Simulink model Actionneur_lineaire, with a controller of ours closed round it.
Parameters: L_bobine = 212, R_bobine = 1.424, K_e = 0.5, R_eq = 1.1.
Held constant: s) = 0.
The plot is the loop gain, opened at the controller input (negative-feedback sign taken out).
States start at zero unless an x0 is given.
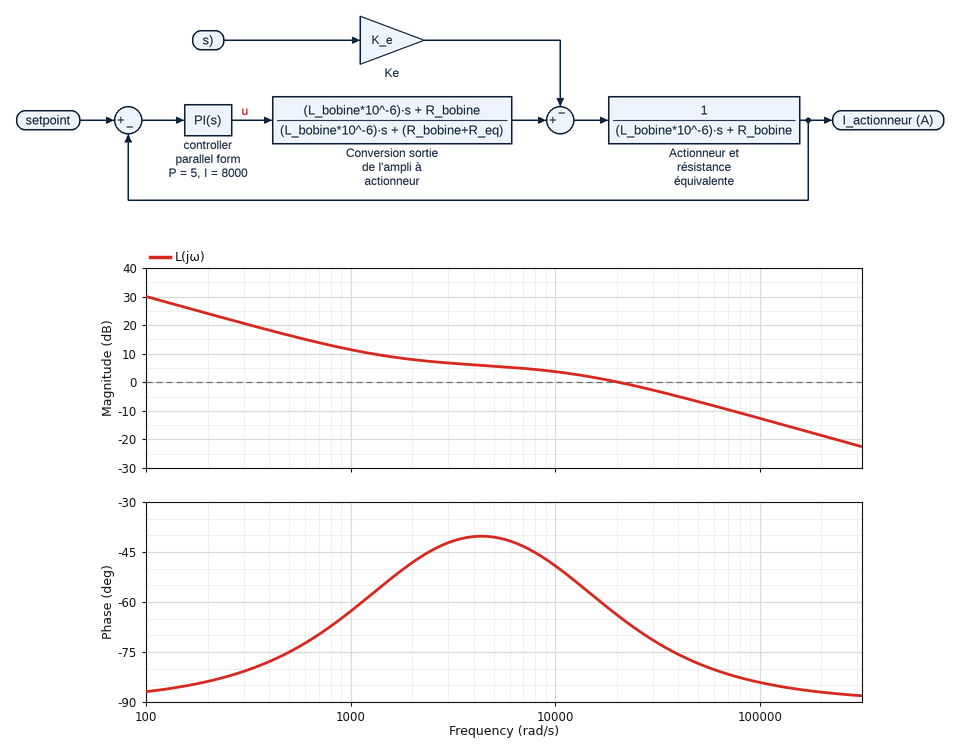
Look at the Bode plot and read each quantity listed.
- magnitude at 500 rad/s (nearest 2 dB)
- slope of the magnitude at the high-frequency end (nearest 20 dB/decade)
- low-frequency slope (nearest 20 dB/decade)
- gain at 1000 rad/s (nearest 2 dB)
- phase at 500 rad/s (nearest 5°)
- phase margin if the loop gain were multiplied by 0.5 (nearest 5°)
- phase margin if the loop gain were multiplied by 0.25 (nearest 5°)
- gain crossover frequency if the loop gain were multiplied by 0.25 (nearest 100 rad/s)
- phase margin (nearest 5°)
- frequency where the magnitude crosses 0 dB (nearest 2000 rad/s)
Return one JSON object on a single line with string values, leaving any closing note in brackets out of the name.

{"magnitude at 500 rad/s": "16 dB", "slope of the magnitude at the high-frequency end": "-20 dB/decade", "low-frequency slope": "-20 dB/decade", "gain at 1000 rad/s": "12 dB", "phase at 500 rad/s": "-75°", "phase margin if the loop gain were multiplied by 0.5": "140°", "phase margin if the loop gain were multiplied by 0.25": "115°", "gain crossover frequency if the loop gain were multiplied by 0.25": "900 rad/s", "phase margin": "115°", "frequency where the magnitude crosses 0 dB": "20000 rad/s"}
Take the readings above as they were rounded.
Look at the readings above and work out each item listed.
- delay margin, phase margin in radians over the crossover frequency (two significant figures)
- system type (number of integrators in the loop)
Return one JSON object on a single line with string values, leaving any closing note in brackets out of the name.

{"delay margin, phase margin in radians over the crossover frequency": "0.00010 s", "system type": "1"}
